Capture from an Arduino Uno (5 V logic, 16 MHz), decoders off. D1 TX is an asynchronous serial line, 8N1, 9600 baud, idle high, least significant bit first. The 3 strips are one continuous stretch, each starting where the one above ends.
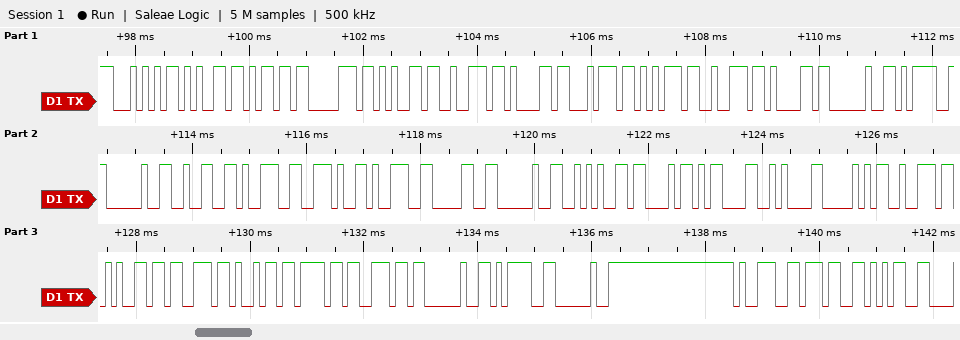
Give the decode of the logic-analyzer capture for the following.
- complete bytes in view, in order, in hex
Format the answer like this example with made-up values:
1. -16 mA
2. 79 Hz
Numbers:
1. 54 65 6D 70 65 72 61 74 75 72 61 20 3D 20 32 39 2E 39 30 20 2A 43 0D 0A 50 72 65 73 69 6F 6E 20 3D 20 39 37 35
